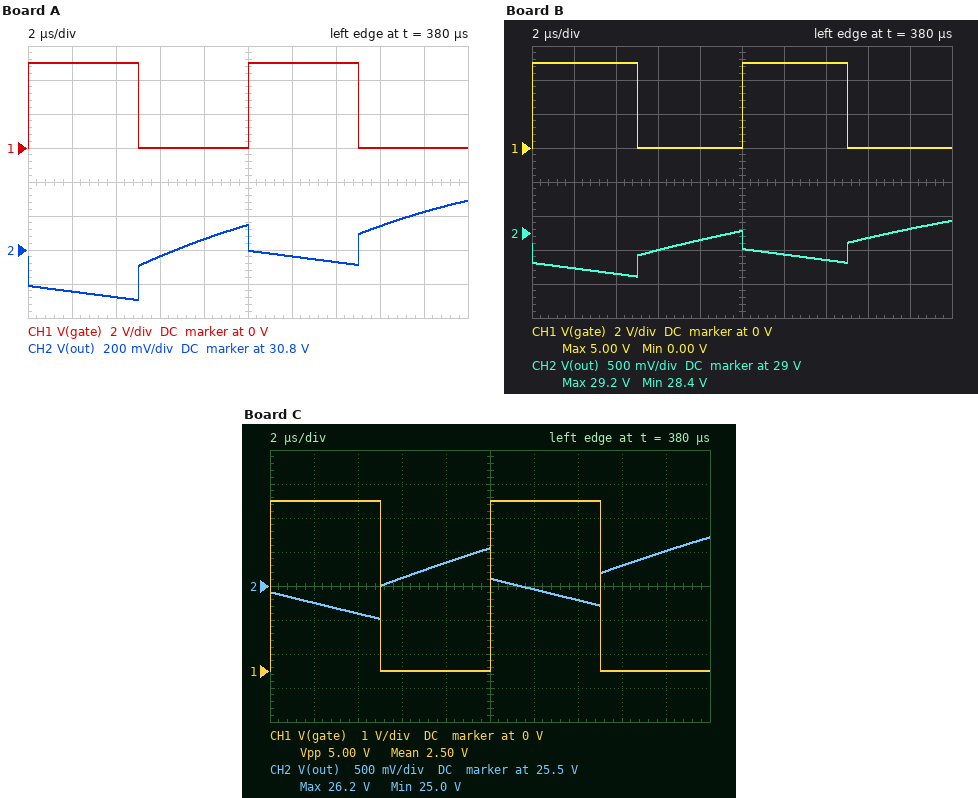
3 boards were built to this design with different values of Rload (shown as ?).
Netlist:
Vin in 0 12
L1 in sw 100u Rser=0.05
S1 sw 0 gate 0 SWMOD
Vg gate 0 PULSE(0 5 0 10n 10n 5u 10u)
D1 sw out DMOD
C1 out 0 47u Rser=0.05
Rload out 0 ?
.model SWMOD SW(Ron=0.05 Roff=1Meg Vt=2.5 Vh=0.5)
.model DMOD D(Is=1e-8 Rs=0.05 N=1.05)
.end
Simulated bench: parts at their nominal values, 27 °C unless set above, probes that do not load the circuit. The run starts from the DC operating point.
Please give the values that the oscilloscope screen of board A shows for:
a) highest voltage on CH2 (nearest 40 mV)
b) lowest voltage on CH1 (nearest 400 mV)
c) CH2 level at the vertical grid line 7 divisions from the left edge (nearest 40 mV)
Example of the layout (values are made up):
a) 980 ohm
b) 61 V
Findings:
a) 31.08 V
b) 0 V
c) 30.72 V
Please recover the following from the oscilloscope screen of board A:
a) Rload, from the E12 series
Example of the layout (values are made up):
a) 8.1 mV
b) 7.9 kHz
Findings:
a) 39 Ω
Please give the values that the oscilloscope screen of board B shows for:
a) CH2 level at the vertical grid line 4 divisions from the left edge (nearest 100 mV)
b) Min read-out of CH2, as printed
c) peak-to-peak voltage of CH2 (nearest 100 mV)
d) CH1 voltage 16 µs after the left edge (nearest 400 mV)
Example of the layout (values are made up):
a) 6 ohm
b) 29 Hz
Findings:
a) 28.9 V
b) 28.4 V
c) 800 mV
d) 0 V
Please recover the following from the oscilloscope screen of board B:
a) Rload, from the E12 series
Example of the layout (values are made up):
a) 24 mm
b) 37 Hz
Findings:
a) 15 Ω
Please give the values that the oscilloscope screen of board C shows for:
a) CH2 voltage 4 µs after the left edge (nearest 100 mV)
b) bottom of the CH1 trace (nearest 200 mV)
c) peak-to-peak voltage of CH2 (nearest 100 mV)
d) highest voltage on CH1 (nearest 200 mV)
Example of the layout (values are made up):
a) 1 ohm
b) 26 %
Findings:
a) 25.1 V
b) 0 V
c) 1.2 V
d) 5.0 V
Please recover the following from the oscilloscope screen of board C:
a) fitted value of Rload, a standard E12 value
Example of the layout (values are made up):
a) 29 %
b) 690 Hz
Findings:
a) 6.8 Ω
